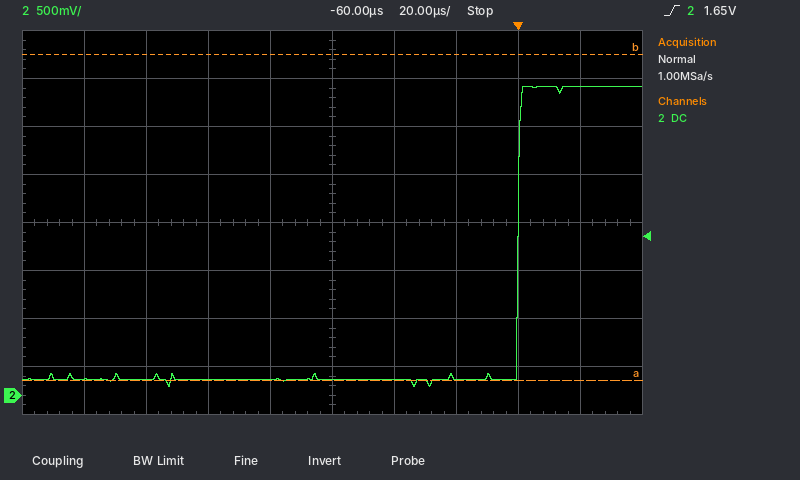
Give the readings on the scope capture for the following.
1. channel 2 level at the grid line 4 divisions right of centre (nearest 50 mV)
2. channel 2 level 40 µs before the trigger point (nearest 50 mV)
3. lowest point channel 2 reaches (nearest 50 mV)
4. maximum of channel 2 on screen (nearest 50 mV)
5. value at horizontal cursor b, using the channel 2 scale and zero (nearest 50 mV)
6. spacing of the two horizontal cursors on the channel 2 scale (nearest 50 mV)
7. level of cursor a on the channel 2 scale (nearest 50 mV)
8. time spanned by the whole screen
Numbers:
3.20 V
150 mV
100 mV
3.20 V
3.55 V
3.40 V
150 mV
200 µs
